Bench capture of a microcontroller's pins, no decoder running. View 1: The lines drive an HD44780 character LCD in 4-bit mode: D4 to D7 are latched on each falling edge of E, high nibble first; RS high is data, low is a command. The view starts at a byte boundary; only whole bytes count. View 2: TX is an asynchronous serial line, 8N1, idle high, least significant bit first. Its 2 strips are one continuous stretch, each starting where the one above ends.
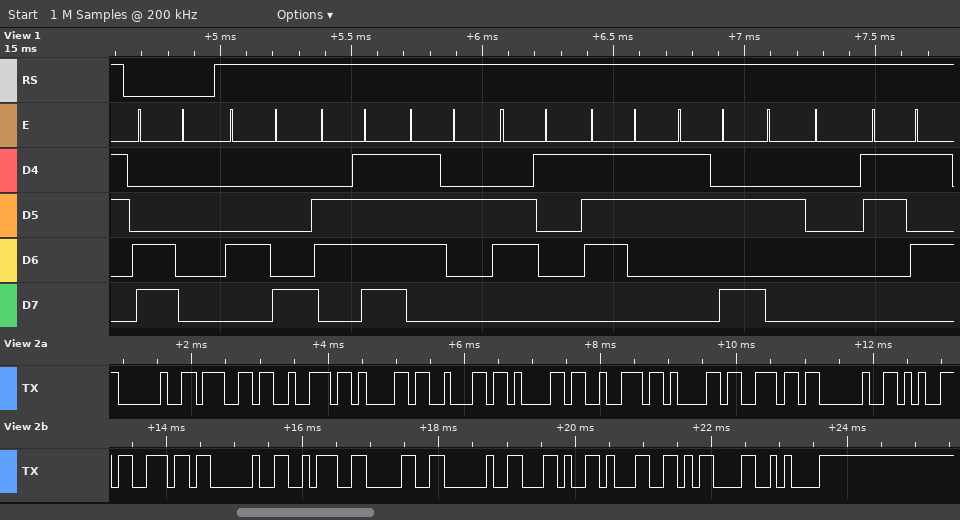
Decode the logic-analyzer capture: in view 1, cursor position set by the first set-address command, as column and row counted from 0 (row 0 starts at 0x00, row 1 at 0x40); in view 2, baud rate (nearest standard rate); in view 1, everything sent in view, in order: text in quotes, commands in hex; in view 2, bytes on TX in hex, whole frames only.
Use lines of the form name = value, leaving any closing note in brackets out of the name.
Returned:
in view 1, cursor position set by the first set-address command, as column and row counted from 0 = column 0, row 1
in view 2, baud rate = 9600 baud
in view 1, everything sent in view, in order: text in quotes, commands in hex = 0xC0 "Horas: 5"
in view 2, bytes on TX in hex, whole frames only = 0x20 0x67 0x72 0x61 0x62 0x61 0x72 0x61 0x6E 0x20 0x65 0x6E 0x20 0x3A 0x30 0x20 0x2C 0x31 0x0D 0x0A
